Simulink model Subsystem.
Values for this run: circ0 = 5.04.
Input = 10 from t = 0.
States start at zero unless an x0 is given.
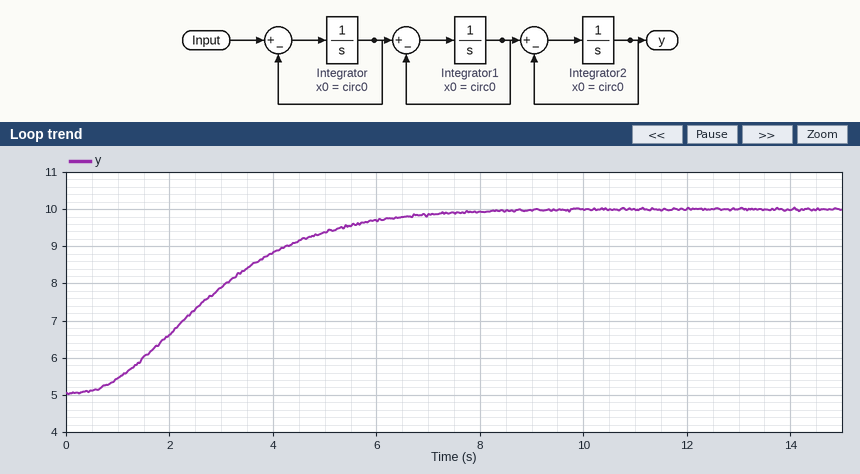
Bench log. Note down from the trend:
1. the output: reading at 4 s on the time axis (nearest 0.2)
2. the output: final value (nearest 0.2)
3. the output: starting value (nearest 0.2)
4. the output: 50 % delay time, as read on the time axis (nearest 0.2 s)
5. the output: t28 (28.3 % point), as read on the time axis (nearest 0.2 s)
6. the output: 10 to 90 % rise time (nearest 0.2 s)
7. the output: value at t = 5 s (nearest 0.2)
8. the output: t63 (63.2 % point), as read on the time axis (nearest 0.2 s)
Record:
8.8
10.0
5.0
2.6 s
1.8 s
4.2 s
9.4
3.2 s
